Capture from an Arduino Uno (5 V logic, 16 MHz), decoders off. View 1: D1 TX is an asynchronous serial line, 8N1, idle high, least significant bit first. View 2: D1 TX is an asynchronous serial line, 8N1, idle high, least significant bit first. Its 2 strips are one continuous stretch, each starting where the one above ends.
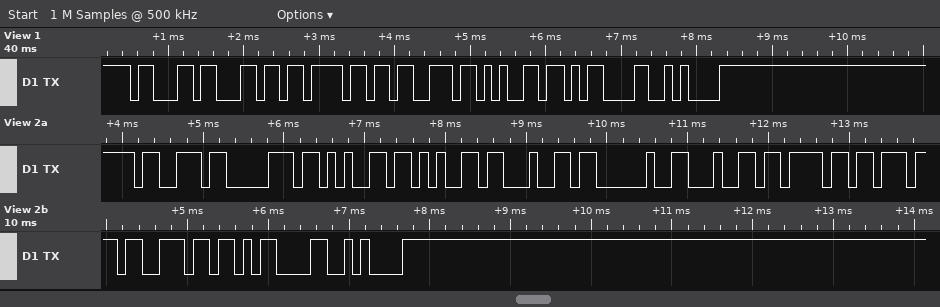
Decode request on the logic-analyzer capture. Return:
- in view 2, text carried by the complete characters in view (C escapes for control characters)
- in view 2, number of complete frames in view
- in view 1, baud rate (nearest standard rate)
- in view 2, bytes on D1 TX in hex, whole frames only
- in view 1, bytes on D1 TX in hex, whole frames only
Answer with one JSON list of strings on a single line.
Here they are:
["\"speed down\\r\\n\"", "12", "9600 baud", "0x73 0x70 0x65 0x65 0x64 0x20 0x64 0x6F 0x77 0x6E 0x0D 0x0A", "63 6C 6F 73 65 0D 0A"]
